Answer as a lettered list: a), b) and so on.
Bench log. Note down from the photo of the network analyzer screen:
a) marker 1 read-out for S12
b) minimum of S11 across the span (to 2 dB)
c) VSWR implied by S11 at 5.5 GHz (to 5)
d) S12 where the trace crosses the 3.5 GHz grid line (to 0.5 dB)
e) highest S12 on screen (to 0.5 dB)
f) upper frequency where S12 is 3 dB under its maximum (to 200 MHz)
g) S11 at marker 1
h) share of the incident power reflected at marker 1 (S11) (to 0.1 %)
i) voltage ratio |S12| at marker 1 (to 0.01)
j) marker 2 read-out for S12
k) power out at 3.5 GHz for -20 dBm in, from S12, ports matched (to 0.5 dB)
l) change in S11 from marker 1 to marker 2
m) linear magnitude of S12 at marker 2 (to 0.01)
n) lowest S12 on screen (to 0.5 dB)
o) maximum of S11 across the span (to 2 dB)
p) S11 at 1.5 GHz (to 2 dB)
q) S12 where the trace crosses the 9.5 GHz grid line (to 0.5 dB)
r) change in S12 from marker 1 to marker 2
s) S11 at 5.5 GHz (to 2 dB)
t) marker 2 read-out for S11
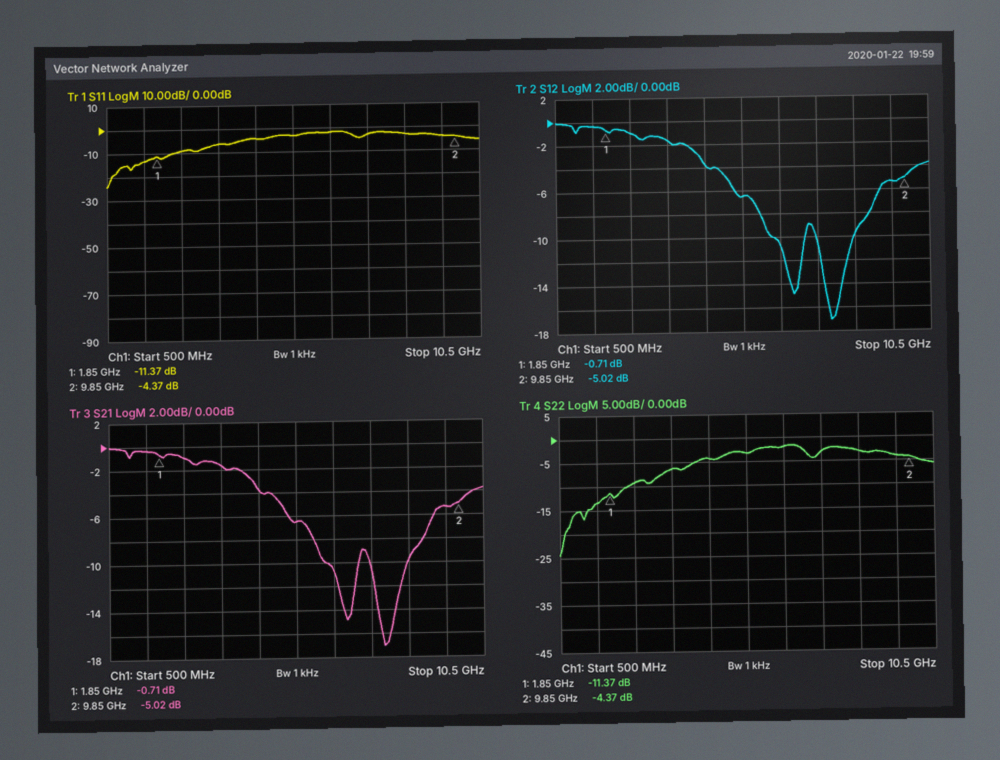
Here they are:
a) -0.71 dB
b) -24 dB
c) 5
d) -1.5 dB
e) 0.0 dB
f) 4.4 GHz
g) -11.37 dB
h) 7.3 %
i) 0.92
j) -5.02 dB
k) -21.5 dBm
l) 7.00 dB
m) 0.56
n) -17.0 dB
o) -2 dB
p) -14 dB
q) -5.5 dB
r) -4.31 dB
s) -4 dB
t) -4.37 dB
